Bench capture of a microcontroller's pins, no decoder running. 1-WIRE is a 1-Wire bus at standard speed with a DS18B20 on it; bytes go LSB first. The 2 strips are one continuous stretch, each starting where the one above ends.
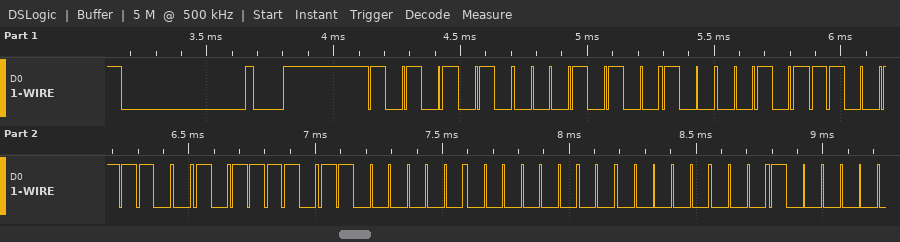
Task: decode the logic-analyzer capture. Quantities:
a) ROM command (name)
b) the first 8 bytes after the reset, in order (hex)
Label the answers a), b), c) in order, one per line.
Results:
a) Match ROM
b) 55 28 A1 73 7A 03 00 00
